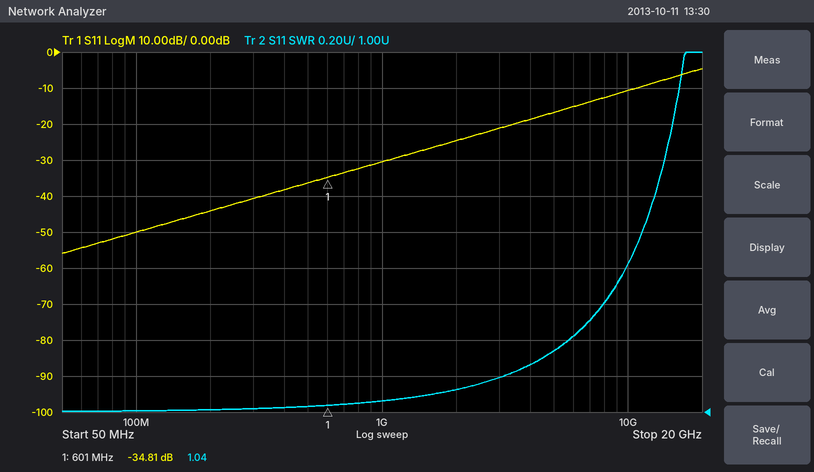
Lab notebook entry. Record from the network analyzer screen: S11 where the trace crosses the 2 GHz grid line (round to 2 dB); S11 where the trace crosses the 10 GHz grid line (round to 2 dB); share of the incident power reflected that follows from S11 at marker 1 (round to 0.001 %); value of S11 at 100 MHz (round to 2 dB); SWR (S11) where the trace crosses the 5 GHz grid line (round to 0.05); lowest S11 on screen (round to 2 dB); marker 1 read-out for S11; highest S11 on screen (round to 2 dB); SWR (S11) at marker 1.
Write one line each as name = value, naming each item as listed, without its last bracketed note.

S11 where the trace crosses the 2 GHz grid line = -24 dB
S11 where the trace crosses the 10 GHz grid line = -10 dB
share of the incident power reflected that follows from S11 at marker 1 = 0.033 %
value of S11 at 100 MHz = -50 dB
SWR (S11) where the trace crosses the 5 GHz grid line = 1.35
lowest S11 on screen = -56 dB
marker 1 read-out for S11 = -34.81 dB
highest S11 on screen = -4 dB
SWR (S11) at marker 1 = 1.04
